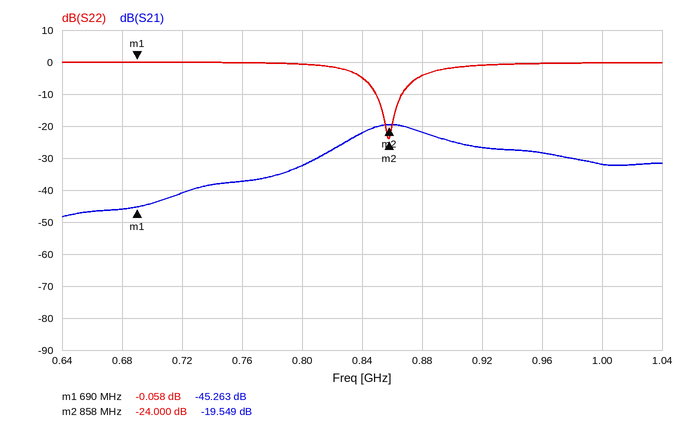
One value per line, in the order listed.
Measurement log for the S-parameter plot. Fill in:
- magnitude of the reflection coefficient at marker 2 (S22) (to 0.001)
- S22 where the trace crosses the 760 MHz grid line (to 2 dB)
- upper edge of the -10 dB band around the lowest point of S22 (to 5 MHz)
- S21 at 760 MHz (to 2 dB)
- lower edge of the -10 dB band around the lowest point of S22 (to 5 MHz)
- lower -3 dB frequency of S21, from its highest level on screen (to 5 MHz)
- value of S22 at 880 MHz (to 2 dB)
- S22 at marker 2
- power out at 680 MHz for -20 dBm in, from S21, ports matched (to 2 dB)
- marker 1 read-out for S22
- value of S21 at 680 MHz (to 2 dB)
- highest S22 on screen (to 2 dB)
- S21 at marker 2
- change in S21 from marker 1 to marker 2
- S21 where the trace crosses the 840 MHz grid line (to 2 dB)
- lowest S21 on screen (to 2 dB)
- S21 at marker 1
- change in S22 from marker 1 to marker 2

0.063
0 dB
865 MHz
-38 dB
850 MHz
840 MHz
-4 dB
-24.000 dB
-66 dBm
-0.058 dB
-46 dB
0 dB
-19.549 dB
25.714 dB
-22 dB
-48 dB
-45.263 dB
-23.942 dB
